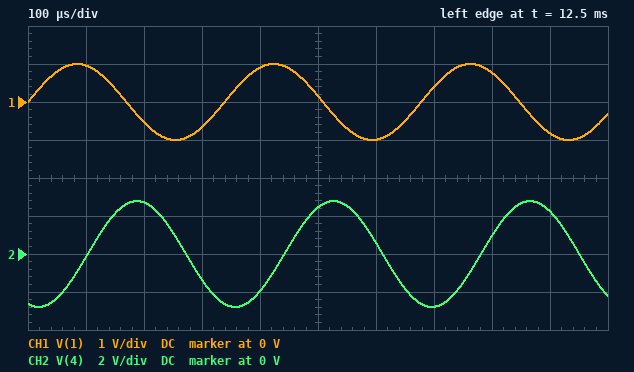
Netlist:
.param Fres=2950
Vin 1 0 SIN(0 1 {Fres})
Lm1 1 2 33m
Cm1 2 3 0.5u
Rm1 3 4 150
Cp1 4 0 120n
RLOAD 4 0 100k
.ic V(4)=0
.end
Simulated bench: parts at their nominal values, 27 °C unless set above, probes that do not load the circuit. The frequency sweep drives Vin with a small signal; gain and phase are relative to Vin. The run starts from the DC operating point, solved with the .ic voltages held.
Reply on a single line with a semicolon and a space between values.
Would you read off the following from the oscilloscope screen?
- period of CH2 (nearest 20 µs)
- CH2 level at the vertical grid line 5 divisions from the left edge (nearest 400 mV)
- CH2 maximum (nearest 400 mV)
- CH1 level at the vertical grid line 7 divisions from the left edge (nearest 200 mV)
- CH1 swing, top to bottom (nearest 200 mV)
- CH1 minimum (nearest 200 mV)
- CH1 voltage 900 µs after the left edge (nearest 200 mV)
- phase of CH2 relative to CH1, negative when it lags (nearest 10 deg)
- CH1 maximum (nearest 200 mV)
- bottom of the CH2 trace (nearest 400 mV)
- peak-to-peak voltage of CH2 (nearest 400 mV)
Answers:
340 µs; 2.4 V; 2.8 V; 400 mV; 2.0 V; -1.0 V; -800 mV; -110 deg; 1.0 V; -2.8 V; 5.6 V
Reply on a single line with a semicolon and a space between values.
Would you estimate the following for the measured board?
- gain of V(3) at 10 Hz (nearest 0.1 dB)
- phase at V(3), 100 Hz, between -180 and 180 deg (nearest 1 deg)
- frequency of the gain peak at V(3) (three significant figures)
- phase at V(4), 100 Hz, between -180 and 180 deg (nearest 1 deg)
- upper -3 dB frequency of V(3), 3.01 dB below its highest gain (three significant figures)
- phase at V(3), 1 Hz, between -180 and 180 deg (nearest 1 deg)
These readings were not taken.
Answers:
-2.1 dB; 2 deg; 2.77 kHz; 1 deg; 3.13 kHz; 69 deg
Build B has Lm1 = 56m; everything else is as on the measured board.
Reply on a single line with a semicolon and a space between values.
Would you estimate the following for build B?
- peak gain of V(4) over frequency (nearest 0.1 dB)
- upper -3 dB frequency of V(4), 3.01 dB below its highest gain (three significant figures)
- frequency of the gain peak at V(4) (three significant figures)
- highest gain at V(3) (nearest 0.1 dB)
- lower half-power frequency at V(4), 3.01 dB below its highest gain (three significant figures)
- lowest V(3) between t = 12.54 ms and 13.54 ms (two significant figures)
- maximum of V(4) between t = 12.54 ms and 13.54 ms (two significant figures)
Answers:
12.1 dB; 2.35 kHz; 2.14 kHz; 12.3 dB; 1.91 kHz; -940 mV; 890 mV
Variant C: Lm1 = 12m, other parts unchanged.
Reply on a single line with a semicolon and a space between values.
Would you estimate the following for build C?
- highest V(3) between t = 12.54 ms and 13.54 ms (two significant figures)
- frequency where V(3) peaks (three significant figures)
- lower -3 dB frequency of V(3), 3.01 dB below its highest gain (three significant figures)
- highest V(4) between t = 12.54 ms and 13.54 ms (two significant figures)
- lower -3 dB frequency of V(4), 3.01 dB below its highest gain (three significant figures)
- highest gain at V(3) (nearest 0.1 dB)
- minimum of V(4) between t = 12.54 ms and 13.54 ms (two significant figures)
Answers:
1.3 V; 4.50 kHz; 3.40 kHz; 1.2 V; 3.27 kHz; 6.7 dB; -1.2 V
